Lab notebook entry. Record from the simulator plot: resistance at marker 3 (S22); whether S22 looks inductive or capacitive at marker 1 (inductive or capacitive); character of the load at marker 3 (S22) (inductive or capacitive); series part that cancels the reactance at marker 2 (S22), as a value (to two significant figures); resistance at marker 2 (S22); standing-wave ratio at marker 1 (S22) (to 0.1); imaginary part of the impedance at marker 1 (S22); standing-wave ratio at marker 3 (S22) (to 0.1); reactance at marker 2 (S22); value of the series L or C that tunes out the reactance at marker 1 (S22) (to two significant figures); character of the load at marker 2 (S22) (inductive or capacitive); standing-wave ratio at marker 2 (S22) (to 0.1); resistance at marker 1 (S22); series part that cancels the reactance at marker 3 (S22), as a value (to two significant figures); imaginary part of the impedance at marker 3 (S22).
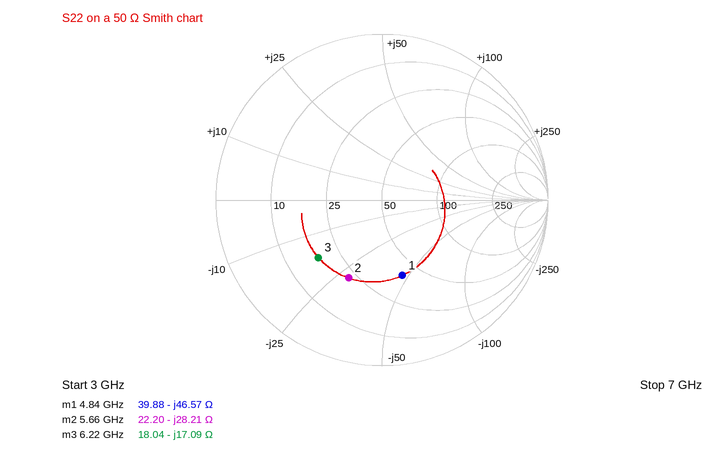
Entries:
18.04 Ω
capacitive
capacitive
790 pH
22.20 Ω
2.8
-46.57 Ω
3.1
-28.21 Ω
1.5 nH
capacitive
3.1
39.88 Ω
440 pH
-17.09 Ω
